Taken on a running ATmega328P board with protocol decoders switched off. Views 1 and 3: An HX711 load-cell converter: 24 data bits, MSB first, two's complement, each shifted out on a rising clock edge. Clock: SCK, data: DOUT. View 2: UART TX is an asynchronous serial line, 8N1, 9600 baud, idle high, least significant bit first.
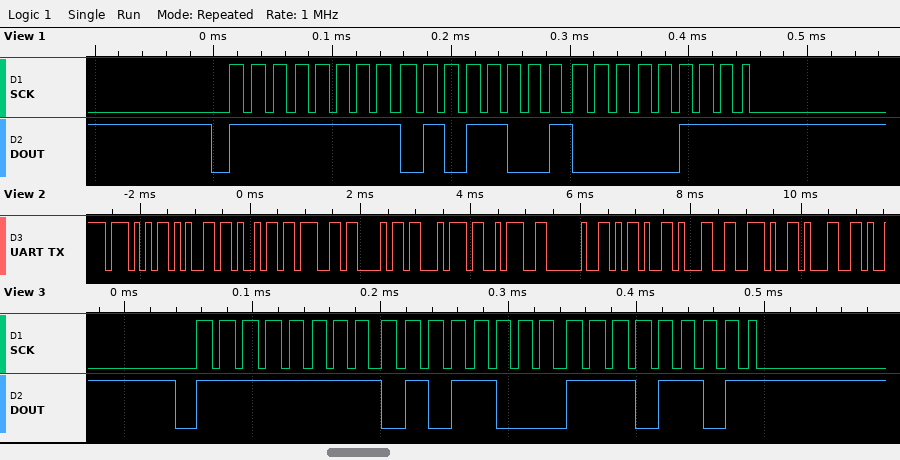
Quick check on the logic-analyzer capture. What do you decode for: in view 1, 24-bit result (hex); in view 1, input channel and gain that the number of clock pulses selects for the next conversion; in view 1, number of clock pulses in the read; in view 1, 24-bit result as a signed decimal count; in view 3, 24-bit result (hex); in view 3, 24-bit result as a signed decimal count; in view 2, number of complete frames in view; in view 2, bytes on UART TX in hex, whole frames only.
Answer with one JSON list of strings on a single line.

["0xFF5907", "channel A, gain 128", "25", "-42745", "0xFF58ED", "-42771", "12", "57 65 69 67 68 74 3A 20 2D 31 2E 31"]
